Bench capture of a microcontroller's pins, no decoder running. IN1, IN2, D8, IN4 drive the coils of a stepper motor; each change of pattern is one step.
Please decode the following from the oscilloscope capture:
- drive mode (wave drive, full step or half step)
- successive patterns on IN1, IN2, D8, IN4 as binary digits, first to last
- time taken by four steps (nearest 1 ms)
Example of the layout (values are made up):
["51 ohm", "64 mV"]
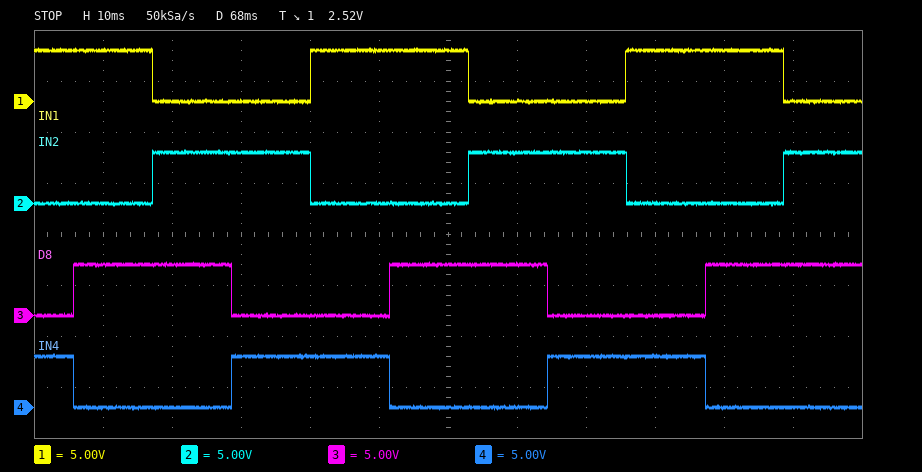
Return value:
["full step", "1001 1010 0110 0101 1001 1010 0110 0101 1001 1010 0110", "46 ms"]
